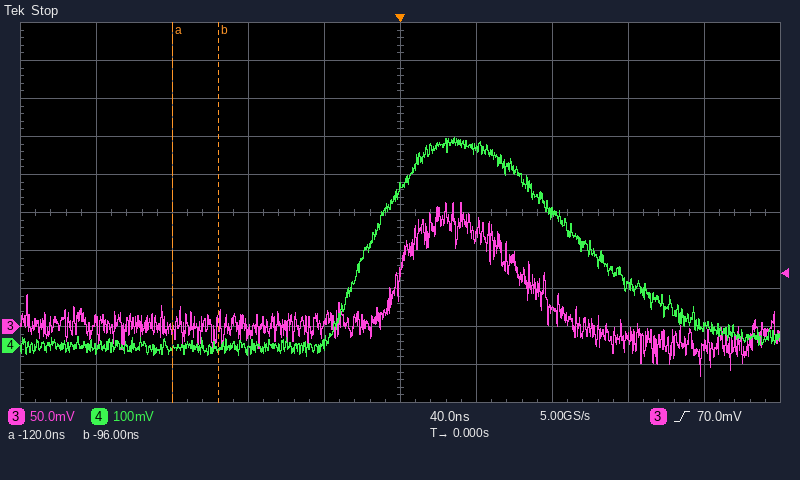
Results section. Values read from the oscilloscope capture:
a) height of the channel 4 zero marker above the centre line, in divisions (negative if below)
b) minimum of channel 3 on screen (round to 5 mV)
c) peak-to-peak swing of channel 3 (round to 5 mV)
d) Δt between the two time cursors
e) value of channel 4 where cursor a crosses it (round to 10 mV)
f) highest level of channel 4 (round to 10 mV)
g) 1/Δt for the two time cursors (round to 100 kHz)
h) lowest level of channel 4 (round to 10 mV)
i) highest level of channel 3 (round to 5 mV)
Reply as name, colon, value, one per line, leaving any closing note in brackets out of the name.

height of the channel 4 zero marker above the centre line, in divisions: -3.5 div
minimum of channel 3 on screen: -65 mV
peak-to-peak swing of channel 3: 230 mV
Δt between the two time cursors: 24 ns
value of channel 4 where cursor a crosses it: -10 mV
highest level of channel 4: 550 mV
1/Δt for the two time cursors: 41.7 MHz
lowest level of channel 4: -30 mV
highest level of channel 3: 165 mV
